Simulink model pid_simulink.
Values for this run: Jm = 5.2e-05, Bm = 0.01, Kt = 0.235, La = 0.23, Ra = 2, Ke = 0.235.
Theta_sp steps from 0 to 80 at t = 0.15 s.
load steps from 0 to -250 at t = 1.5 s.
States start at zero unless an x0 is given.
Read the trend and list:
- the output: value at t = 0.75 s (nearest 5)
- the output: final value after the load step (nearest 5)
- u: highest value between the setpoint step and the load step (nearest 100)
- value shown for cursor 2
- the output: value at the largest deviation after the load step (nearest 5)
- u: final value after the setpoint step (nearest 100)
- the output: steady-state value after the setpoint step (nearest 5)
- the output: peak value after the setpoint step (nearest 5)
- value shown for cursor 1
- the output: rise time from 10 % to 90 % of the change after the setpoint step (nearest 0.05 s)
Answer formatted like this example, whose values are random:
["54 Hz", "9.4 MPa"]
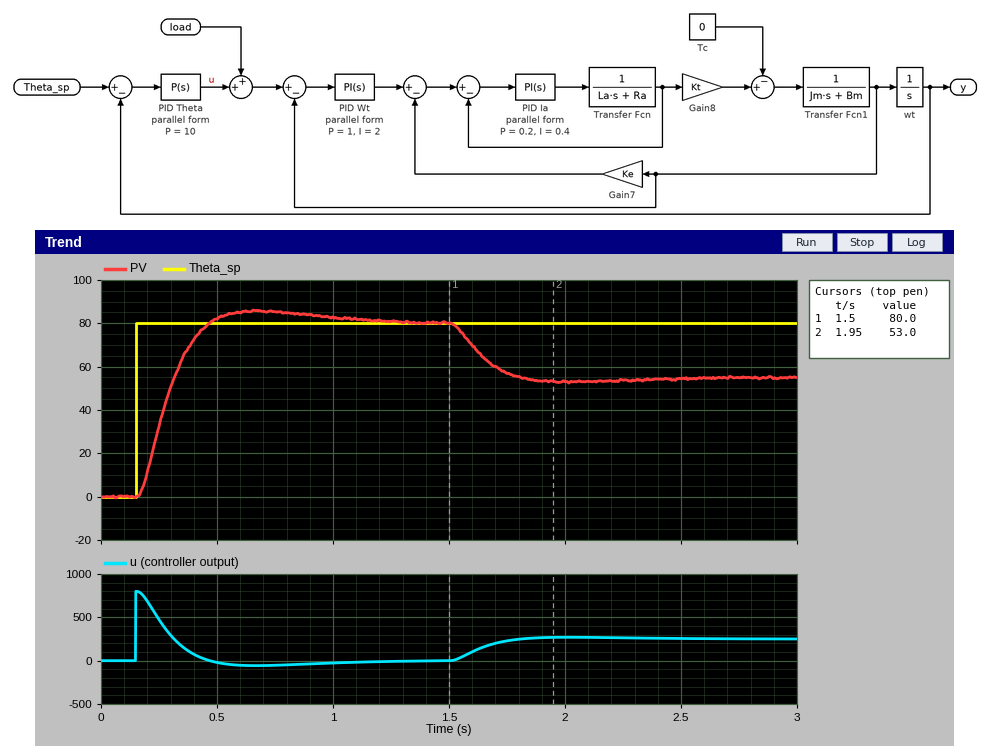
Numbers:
["85", "55", "800", "53.0", "55", "0", "80", "85", "80.0", "0.20 s"]
